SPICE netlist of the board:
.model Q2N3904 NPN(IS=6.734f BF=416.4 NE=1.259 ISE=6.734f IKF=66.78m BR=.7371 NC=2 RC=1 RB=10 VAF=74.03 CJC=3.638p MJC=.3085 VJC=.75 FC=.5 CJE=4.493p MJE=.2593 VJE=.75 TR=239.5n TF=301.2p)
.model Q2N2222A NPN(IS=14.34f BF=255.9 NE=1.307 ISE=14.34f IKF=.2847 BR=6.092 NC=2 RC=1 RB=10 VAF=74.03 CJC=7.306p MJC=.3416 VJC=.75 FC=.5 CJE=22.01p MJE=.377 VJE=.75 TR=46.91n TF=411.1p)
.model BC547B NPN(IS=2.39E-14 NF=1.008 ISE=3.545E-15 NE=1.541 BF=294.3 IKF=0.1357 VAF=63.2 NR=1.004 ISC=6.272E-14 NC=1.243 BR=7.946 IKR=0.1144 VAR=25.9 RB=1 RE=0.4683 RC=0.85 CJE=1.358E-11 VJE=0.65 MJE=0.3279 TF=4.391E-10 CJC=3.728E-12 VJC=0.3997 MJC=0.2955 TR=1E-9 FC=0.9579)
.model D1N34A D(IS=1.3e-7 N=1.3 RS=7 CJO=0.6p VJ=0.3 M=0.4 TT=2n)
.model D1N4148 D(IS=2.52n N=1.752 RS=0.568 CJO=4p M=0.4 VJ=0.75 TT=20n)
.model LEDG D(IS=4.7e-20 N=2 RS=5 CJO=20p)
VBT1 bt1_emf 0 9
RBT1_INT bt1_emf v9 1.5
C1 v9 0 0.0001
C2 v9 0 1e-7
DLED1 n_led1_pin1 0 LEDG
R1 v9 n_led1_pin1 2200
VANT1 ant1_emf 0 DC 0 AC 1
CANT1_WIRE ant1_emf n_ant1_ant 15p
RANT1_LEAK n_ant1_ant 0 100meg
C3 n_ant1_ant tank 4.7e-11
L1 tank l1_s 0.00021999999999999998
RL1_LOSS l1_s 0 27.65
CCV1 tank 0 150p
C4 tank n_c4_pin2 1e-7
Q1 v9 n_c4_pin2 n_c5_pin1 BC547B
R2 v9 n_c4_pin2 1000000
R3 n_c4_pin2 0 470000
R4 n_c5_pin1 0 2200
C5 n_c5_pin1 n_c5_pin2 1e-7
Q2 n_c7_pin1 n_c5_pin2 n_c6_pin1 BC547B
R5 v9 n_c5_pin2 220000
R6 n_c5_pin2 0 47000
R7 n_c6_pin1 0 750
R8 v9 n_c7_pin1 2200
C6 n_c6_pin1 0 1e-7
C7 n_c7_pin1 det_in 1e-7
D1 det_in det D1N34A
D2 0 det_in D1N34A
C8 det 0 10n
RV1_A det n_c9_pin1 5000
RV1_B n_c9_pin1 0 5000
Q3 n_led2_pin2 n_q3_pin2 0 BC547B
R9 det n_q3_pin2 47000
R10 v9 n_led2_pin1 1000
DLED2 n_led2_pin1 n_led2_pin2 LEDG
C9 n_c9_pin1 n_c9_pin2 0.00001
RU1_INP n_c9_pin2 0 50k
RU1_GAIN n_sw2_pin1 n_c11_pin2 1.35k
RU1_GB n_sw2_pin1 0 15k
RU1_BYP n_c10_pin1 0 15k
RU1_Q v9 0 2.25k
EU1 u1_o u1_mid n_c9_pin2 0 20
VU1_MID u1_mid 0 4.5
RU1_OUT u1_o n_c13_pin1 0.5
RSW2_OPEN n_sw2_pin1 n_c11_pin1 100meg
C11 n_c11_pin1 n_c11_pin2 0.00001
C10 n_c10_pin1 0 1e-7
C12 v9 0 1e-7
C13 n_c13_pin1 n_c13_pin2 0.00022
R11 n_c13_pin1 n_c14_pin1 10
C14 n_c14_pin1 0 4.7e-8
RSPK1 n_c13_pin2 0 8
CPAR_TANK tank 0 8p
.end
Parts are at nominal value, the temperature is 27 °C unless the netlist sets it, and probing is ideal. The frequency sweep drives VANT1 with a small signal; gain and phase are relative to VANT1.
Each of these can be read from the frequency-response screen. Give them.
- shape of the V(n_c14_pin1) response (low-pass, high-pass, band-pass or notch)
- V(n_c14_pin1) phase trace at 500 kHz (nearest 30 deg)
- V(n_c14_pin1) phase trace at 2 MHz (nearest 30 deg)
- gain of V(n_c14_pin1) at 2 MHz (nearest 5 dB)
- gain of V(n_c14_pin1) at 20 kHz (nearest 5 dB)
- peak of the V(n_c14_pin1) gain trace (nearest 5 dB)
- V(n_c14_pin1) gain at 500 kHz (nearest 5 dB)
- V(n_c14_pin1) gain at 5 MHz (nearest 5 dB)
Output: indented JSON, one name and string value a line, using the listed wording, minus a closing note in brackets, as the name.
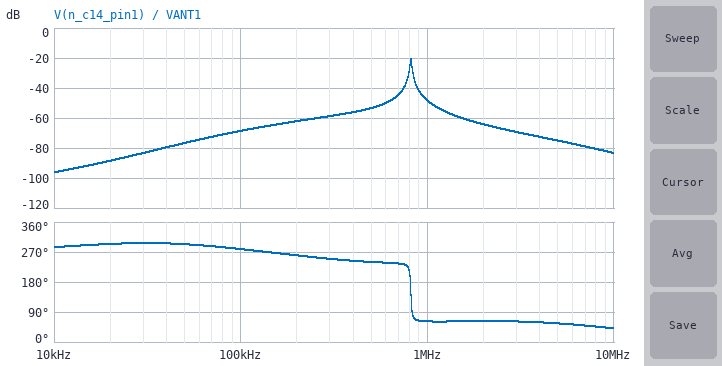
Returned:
{
  "shape of the V(n_c14_pin1) response": "band-pass",
  "V(n_c14_pin1) phase trace at 500 kHz": "240 deg",
  "V(n_c14_pin1) phase trace at 2 MHz": "60 deg",
  "gain of V(n_c14_pin1) at 2 MHz": "-65 dB",
  "gain of V(n_c14_pin1) at 20 kHz": "-90 dB",
  "peak of the V(n_c14_pin1) gain trace": "-20 dB",
  "V(n_c14_pin1) gain at 500 kHz": "-55 dB",
  "V(n_c14_pin1) gain at 5 MHz": "-75 dB"
}
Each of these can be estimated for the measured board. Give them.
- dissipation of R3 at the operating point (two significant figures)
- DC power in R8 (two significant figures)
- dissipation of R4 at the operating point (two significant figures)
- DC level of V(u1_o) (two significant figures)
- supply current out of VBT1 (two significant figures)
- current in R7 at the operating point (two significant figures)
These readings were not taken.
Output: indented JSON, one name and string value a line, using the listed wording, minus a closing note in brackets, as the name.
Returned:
{
  "dissipation of R3 at the operating point": "10 µW",
  "DC power in R8": "2.5 mW",
  "dissipation of R4 at the operating point": "1.1 mW",
  "DC level of V(u1_o)": "4.5 V",
  "supply current out of VBT1": "9.0 mA",
  "current in R7 at the operating point": "1.1 mA"
}
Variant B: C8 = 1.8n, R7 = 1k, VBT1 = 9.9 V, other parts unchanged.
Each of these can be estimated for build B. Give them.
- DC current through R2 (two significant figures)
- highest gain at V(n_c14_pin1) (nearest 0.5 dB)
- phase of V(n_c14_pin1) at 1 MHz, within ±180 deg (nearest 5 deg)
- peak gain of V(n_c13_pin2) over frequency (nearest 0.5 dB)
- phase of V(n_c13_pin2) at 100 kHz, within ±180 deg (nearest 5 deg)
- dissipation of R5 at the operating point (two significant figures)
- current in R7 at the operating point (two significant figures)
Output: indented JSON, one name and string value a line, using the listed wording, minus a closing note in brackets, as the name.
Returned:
{
  "DC current through R2": "7.5 µA",
  "highest gain at V(n_c14_pin1)": "-7.5 dB",
  "phase of V(n_c14_pin1) at 1 MHz, within ±180 deg": "65 deg",
  "peak gain of V(n_c13_pin2) over frequency": "1.0 dB",
  "phase of V(n_c13_pin2) at 100 kHz, within ±180 deg": "-60 deg",
  "dissipation of R5 at the operating point": "310 µW",
  "current in R7 at the operating point": "980 µA"
}
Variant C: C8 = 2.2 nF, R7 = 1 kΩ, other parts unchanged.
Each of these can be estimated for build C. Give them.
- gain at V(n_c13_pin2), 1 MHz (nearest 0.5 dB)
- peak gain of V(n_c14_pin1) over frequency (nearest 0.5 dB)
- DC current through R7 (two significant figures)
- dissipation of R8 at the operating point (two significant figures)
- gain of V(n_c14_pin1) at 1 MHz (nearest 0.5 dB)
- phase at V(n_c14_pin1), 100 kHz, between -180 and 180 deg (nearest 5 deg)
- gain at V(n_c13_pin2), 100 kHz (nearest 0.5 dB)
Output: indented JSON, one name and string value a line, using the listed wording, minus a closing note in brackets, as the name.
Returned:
{
  "gain at V(n_c13_pin2), 1 MHz": "-27.5 dB",
  "peak gain of V(n_c14_pin1) over frequency": "-10.5 dB",
  "DC current through R7": "840 µA",
  "dissipation of R8 at the operating point": "1.6 mW",
  "gain of V(n_c14_pin1) at 1 MHz": "-37.0 dB",
  "phase at V(n_c14_pin1), 100 kHz, between -180 and 180 deg": "-85 deg",
  "gain at V(n_c13_pin2), 100 kHz": "-56.5 dB"
}
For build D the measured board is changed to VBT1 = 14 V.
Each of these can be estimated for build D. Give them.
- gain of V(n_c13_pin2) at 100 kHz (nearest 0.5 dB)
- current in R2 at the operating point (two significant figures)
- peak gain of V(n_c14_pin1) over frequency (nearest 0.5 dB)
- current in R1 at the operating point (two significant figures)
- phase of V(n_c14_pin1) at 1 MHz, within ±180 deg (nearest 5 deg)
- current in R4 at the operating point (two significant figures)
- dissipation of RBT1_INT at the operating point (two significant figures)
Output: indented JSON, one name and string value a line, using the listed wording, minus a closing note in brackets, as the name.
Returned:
{
  "gain of V(n_c13_pin2) at 100 kHz": "-65.0 dB",
  "current in R2 at the operating point": "11 µA",
  "peak gain of V(n_c14_pin1) over frequency": "-14.5 dB",
  "current in R1 at the operating point": "5.4 mA",
  "phase of V(n_c14_pin1) at 1 MHz, within ±180 deg": "65 deg",
  "current in R4 at the operating point": "1.2 mA",
  "dissipation of RBT1_INT at the operating point": "340 µW"
}
